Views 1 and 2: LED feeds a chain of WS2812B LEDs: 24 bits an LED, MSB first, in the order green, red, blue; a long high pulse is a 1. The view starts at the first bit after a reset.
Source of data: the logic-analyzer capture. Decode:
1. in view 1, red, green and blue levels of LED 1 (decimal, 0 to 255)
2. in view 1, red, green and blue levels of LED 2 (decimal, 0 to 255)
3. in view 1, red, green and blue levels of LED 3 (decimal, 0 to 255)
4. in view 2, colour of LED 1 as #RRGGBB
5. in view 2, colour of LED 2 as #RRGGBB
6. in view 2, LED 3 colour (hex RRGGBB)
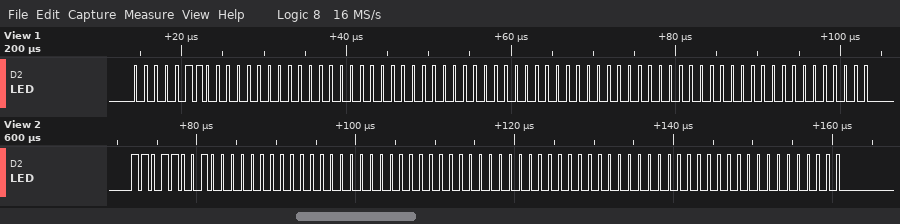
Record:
0, 6, 0
0, 0, 0
0, 0, 0
#00D900
#000000
#000000
